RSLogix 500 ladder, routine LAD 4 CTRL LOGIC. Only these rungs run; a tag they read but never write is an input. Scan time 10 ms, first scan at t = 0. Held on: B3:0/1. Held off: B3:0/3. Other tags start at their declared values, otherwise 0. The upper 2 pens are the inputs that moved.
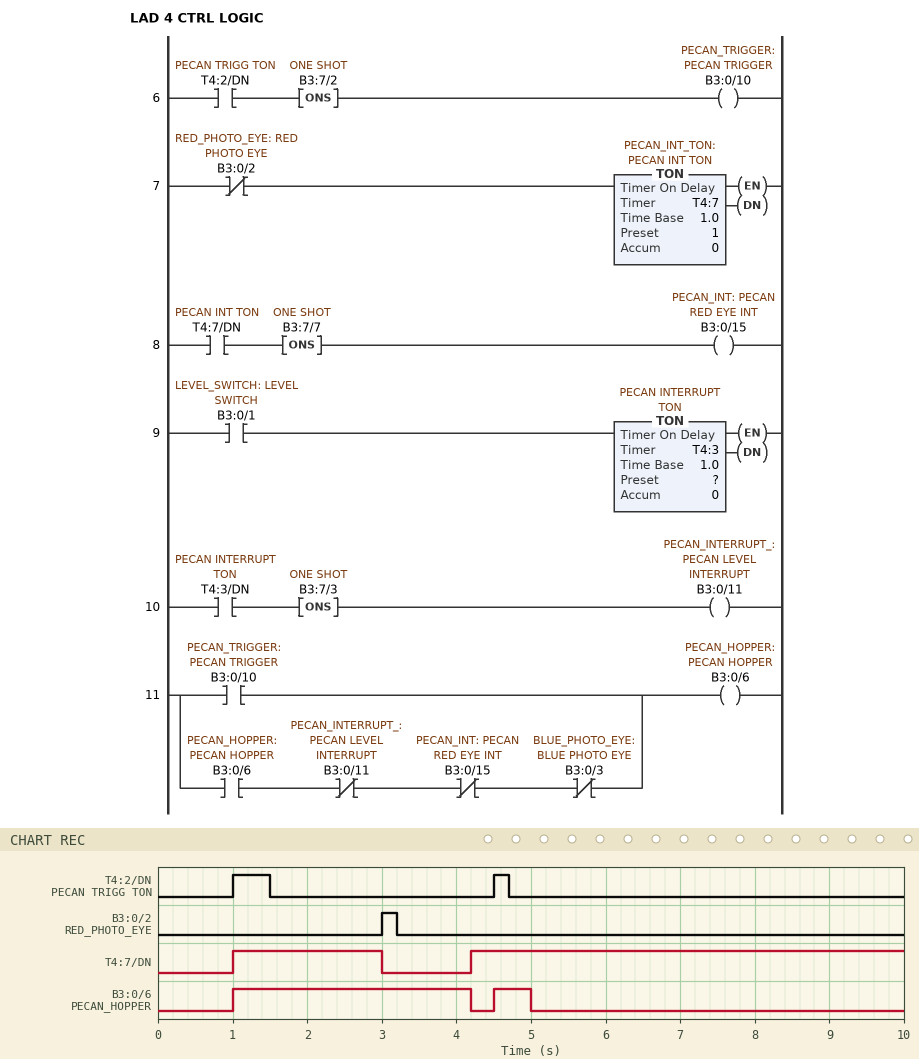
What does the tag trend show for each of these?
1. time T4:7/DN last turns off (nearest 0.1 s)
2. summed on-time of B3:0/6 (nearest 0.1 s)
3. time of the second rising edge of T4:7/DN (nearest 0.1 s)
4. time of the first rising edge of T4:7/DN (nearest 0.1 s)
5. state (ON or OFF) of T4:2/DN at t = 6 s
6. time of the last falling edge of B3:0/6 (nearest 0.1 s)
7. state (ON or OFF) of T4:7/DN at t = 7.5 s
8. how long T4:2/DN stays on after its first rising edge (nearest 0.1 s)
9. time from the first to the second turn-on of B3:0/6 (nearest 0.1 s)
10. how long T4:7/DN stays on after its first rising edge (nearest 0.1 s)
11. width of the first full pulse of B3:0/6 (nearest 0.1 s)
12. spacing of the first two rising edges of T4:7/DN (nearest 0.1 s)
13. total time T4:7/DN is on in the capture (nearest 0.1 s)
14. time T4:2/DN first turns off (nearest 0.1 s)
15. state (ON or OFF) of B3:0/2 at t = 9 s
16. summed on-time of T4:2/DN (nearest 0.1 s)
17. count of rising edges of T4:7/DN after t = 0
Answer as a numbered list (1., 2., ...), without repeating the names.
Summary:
1. 3.0 s
2. 3.7 s
3. 4.2 s
4. 1.0 s
5. OFF
6. 5.0 s
7. ON
8. 0.5 s
9. 3.5 s
10. 2.0 s
11. 3.2 s
12. 3.2 s
13. 7.8 s
14. 1.5 s
15. OFF
16. 0.7 s
17. 2
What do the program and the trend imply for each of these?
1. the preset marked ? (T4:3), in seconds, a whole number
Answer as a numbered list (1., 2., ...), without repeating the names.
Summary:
1. 5 s
